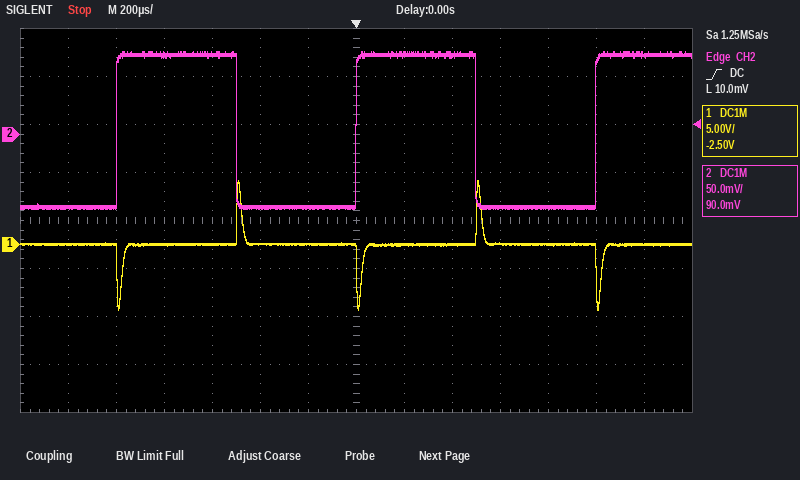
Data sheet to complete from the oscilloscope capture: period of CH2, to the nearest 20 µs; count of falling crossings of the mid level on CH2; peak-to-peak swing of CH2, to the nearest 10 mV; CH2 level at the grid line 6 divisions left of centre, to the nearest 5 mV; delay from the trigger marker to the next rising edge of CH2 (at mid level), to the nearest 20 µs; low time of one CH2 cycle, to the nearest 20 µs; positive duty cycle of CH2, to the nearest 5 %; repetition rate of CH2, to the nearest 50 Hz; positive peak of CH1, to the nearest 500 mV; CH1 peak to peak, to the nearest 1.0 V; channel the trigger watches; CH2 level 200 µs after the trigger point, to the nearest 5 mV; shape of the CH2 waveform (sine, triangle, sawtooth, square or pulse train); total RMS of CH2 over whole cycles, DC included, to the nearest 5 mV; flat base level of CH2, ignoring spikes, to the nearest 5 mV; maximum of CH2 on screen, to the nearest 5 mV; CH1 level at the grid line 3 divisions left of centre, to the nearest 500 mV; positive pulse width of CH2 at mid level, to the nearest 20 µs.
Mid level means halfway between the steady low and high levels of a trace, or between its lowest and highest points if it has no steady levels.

1.00 ms
2
160 mV
-75 mV
1.00 ms
500 µs
50 %
1.00 kHz
6.5 V
13.0 V
CH2
85 mV
square
80 mV
-75 mV
85 mV
0.0 V
500 µs
